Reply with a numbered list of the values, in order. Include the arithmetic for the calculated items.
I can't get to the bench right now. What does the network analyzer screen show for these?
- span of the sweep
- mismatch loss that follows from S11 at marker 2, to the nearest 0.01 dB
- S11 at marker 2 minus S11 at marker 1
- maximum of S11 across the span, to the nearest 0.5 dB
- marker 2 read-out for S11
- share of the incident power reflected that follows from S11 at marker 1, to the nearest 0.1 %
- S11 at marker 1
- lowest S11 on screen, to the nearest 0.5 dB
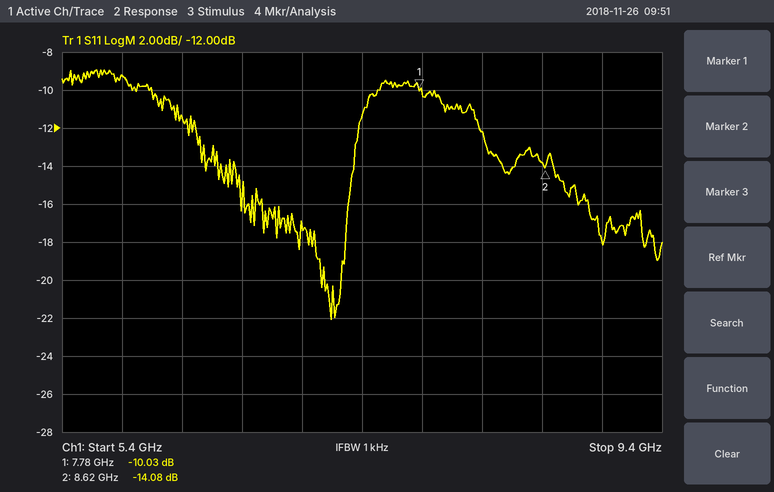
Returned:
1. 4 GHz
2. −10 log10(1 − 10^(-14.08/10)) ≈ 0.17 dB
3. -14.08 − (-10.03) = -4.05 dB
4. -9.0 dB
5. -14.08 dB
6. 10^(-10.03/10) ≈ 9.9 %
7. -10.03 dB
8. -22.0 dB
